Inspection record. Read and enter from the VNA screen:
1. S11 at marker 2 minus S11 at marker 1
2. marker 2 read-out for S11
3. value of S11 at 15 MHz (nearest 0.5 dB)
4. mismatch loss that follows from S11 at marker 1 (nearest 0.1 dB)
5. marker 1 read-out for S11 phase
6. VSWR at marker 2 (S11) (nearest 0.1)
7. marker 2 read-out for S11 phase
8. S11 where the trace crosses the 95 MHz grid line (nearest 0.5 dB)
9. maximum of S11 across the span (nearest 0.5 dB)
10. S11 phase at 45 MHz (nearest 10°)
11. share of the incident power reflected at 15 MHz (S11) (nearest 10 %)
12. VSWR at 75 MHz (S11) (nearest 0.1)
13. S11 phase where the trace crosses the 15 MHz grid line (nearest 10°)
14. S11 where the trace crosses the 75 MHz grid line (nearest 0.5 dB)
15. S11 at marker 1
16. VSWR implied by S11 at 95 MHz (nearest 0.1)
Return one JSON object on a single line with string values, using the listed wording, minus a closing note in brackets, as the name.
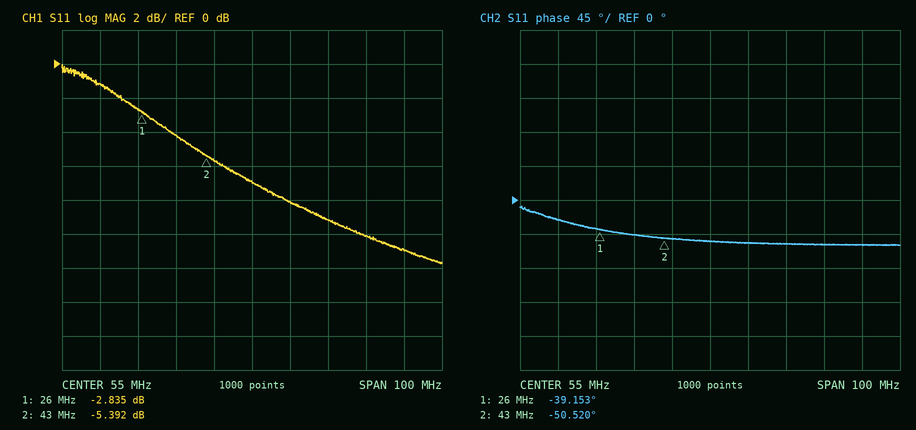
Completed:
{"S11 at marker 2 minus S11 at marker 1": "-2.557 dB", "marker 2 read-out for S11": "-5.392 dB", "value of S11 at 15 MHz": "-1.0 dB", "mismatch loss that follows from S11 at marker 1": "3.2 dB", "marker 1 read-out for S11 phase": "-39.153°", "VSWR at marker 2 (S11)": "3.3", "marker 2 read-out for S11 phase": "-50.520°", "S11 where the trace crosses the 95 MHz grid line": "-11.0 dB", "maximum of S11 across the span": "0.0 dB", "S11 phase at 45 MHz": "-50°", "share of the incident power reflected at 15 MHz (S11)": "80 %", "VSWR at 75 MHz (S11)": "2.1", "S11 phase where the trace crosses the 15 MHz grid line": "-30°", "S11 where the trace crosses the 75 MHz grid line": "-9.0 dB", "S11 at marker 1": "-2.835 dB", "VSWR implied by S11 at 95 MHz": "1.8"}
